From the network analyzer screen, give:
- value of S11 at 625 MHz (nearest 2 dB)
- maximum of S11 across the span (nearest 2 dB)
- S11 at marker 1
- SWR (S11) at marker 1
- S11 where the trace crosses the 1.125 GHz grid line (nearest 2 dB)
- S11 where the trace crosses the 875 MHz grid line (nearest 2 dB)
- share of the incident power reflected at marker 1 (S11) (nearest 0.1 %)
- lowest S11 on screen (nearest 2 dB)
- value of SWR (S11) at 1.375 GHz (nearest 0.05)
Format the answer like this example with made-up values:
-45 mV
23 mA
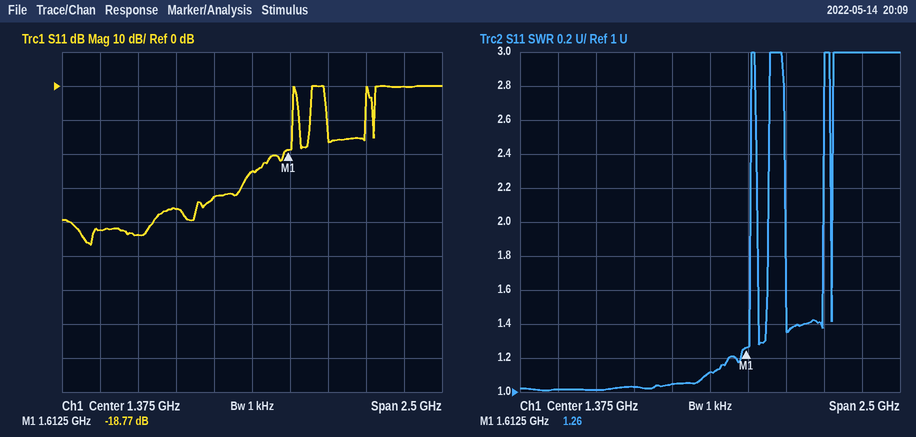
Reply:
-44 dB
0 dB
-18.77 dB
1.26
-32 dB
-36 dB
1.3 %
-46 dB
1.10
